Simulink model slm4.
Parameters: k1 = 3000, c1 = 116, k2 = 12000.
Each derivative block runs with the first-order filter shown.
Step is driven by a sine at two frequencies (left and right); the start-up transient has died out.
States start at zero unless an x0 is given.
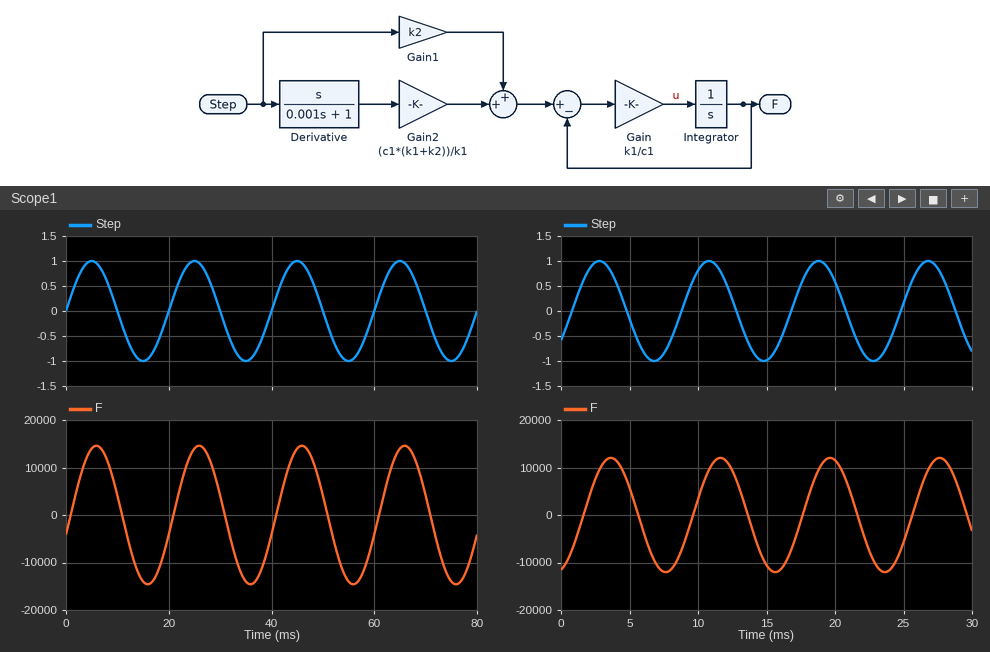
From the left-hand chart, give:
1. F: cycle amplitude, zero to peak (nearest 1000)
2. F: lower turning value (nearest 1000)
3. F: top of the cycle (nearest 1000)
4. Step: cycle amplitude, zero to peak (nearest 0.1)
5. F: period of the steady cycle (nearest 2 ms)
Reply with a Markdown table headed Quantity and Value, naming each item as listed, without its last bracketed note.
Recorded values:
| Quantity | Value |
|---|---|
| F: cycle amplitude, zero to peak | 15000 |
| F: lower turning value | -15000 |
| F: top of the cycle | 15000 |
| Step: cycle amplitude, zero to peak | 1.0 |
| F: period of the steady cycle | 20 ms |
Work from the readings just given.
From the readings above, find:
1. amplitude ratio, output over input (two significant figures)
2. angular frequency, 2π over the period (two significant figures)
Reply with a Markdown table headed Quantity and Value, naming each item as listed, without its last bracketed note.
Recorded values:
| Quantity | Value |
|---|---|
| amplitude ratio, output over input | 15000 |
| angular frequency, 2π over the period | 0.31 rad/ms |
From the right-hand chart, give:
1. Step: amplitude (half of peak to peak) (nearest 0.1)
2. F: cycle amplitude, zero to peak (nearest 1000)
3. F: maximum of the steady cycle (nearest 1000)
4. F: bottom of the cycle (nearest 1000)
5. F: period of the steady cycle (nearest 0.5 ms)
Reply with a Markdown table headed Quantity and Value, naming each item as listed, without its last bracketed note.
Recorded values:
| Quantity | Value |
|---|---|
| Step: amplitude (half of peak to peak) | 1.0 |
| F: cycle amplitude, zero to peak | 12000 |
| F: maximum of the steady cycle | 12000 |
| F: bottom of the cycle | -12000 |
| F: period of the steady cycle | 8.0 ms |
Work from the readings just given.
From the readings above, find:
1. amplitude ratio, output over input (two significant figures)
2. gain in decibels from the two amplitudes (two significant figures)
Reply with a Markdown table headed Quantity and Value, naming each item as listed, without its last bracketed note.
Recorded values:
| Quantity | Value |
|---|---|
| amplitude ratio, output over input | 12000 |
| gain in decibels from the two amplitudes | 82 dB |
